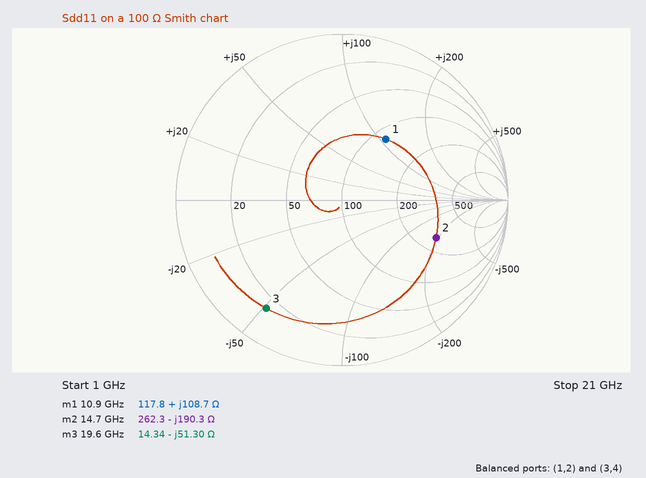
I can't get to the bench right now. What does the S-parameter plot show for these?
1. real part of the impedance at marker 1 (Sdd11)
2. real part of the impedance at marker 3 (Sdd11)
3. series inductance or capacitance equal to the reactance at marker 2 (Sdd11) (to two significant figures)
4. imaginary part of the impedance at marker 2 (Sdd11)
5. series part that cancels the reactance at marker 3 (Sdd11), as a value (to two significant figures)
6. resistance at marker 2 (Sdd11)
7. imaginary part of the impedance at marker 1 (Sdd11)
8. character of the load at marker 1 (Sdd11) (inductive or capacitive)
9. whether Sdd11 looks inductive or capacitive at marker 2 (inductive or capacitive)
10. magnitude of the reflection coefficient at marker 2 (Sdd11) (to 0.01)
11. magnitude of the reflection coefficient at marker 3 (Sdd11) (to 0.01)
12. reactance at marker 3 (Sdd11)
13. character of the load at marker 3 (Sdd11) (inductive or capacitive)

117.8 Ω
14.34 Ω
57 fF
-190.3 Ω
420 pH
262.3 Ω
+108.7 Ω
inductive
capacitive
0.61
0.80
-51.30 Ω
capacitive
